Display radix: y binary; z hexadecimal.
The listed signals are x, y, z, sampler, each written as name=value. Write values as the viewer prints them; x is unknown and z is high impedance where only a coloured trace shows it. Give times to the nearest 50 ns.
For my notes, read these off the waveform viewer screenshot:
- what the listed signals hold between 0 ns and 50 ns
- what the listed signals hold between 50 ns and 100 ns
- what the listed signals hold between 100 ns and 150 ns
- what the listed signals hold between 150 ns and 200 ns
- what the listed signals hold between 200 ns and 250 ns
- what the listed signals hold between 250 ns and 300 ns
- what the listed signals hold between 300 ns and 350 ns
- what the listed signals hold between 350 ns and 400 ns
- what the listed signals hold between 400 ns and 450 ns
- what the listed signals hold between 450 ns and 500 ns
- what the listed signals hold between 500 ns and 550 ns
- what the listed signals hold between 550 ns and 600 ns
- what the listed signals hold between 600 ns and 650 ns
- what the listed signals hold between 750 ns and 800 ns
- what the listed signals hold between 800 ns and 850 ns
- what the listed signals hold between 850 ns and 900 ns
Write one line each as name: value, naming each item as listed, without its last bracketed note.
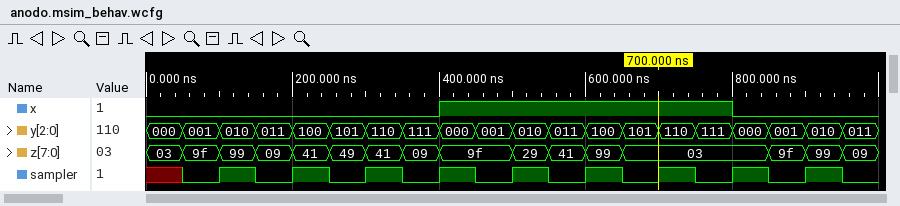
what the listed signals hold between 0 ns and 50 ns: x=0, y=000, z=03, sampler=x
what the listed signals hold between 50 ns and 100 ns: x=0, y=001, z=9f, sampler=0
what the listed signals hold between 100 ns and 150 ns: x=0, y=010, z=99, sampler=1
what the listed signals hold between 150 ns and 200 ns: x=0, y=011, z=09, sampler=0
what the listed signals hold between 200 ns and 250 ns: x=0, y=100, z=41, sampler=1
what the listed signals hold between 250 ns and 300 ns: x=0, y=101, z=49, sampler=0
what the listed signals hold between 300 ns and 350 ns: x=0, y=110, z=41, sampler=1
what the listed signals hold between 350 ns and 400 ns: x=0, y=111, z=09, sampler=0
what the listed signals hold between 400 ns and 450 ns: x=1, y=000, z=9f, sampler=1
what the listed signals hold between 450 ns and 500 ns: x=1, y=001, z=9f, sampler=0
what the listed signals hold between 500 ns and 550 ns: x=1, y=010, z=29, sampler=1
what the listed signals hold between 550 ns and 600 ns: x=1, y=011, z=41, sampler=0
what the listed signals hold between 600 ns and 650 ns: x=1, y=100, z=99, sampler=1
what the listed signals hold between 750 ns and 800 ns: x=1, y=111, z=03, sampler=0
what the listed signals hold between 800 ns and 850 ns: x=0, y=000, z=03, sampler=1
what the listed signals hold between 850 ns and 900 ns: x=0, y=001, z=9f, sampler=0
